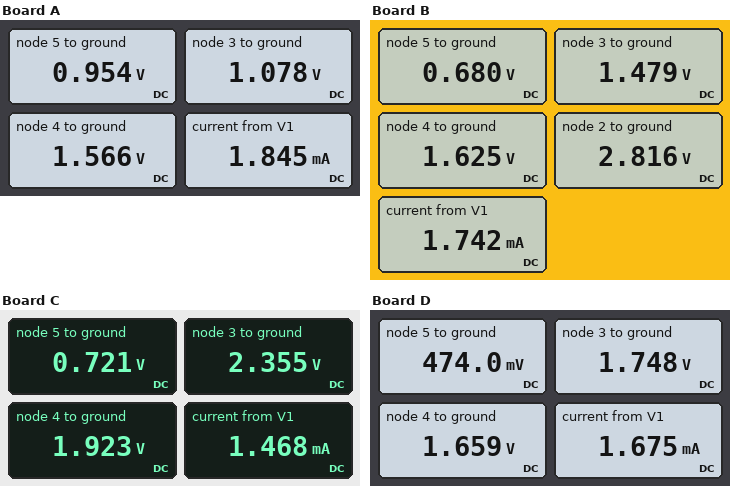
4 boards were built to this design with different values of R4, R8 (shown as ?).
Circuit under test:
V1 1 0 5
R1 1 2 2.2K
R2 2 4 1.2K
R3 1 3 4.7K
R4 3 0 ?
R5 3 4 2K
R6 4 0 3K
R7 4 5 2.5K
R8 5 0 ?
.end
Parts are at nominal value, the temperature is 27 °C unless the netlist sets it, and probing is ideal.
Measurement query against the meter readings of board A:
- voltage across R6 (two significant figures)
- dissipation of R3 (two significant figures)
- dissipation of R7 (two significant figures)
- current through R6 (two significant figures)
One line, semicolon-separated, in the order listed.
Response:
1.6 V; 3.3 mW; 150 µW; 520 µA
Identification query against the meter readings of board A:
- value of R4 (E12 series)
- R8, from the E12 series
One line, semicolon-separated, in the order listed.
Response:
1 kΩ; 3.9 kΩ
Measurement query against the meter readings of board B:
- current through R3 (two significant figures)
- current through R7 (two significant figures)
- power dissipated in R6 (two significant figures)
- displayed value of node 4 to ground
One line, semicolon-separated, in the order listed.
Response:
750 µA; 380 µA; 880 µW; 1.625 V
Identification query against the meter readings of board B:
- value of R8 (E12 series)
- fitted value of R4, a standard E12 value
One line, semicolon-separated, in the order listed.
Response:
1.8 kΩ; 1.8 kΩ
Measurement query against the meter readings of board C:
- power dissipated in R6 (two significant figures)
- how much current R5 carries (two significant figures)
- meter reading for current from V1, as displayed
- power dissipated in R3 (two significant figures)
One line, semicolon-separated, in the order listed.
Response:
1.2 mW; 220 µA; 1.468 mA; 1.5 mW
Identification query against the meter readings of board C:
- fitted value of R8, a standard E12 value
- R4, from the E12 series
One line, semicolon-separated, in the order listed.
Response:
1.5 kΩ; 6.8 kΩ
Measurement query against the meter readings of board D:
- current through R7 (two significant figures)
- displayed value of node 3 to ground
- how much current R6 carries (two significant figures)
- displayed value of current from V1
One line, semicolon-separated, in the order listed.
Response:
470 µA; 1.748 V; 550 µA; 1.675 mA
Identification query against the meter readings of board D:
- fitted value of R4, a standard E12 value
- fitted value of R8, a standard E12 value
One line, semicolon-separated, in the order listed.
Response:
2.7 kΩ; 1 kΩ
